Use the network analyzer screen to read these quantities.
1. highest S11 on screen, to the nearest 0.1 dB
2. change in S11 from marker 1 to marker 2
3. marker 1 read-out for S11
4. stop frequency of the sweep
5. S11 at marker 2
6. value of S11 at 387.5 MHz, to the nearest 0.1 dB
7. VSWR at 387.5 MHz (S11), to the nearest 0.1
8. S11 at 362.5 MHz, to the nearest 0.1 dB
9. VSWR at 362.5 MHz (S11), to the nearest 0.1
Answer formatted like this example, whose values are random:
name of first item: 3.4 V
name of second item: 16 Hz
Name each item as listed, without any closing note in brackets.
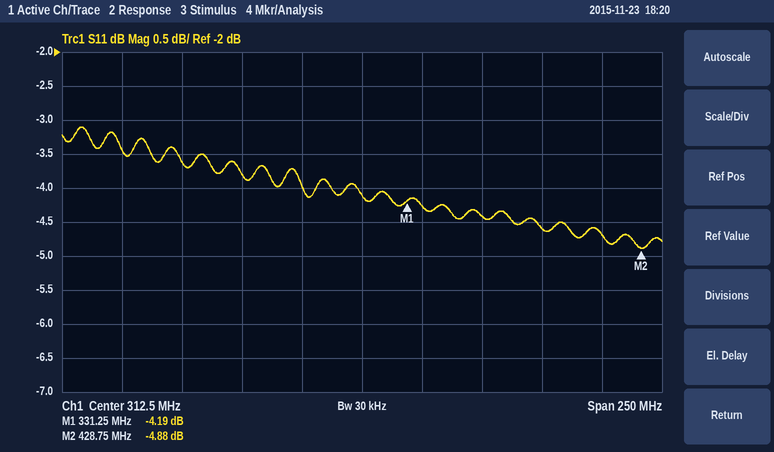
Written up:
highest S11 on screen, to the nearest 0.1 dB: -3.1 dB
change in S11 from marker 1 to marker 2: -0.69 dB
marker 1 read-out for S11: -4.19 dB
stop frequency of the sweep: 437.5 MHz
S11 at marker 2: -4.88 dB
value of S11 at 387.5 MHz, to the nearest 0.1 dB: -4.6 dB
VSWR at 387.5 MHz (S11), to the nearest 0.1: 3.9
S11 at 362.5 MHz, to the nearest 0.1 dB: -4.4 dB
VSWR at 362.5 MHz (S11), to the nearest 0.1: 4.0
